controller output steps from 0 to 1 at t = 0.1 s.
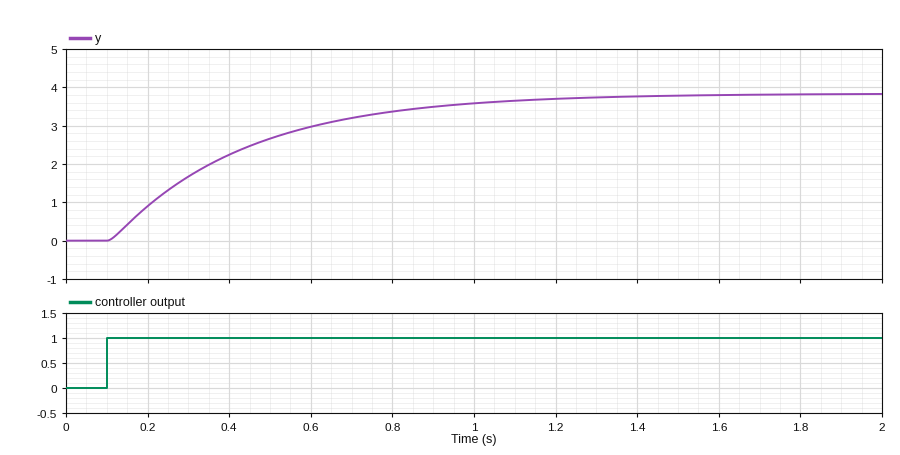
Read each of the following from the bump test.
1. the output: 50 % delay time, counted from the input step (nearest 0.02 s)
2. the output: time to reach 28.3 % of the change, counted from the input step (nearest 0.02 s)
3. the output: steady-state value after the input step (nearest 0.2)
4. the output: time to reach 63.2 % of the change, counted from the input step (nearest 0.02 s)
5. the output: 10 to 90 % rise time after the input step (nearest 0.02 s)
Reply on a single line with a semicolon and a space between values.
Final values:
0.24 s; 0.12 s; 3.8; 0.34 s; 0.72 s
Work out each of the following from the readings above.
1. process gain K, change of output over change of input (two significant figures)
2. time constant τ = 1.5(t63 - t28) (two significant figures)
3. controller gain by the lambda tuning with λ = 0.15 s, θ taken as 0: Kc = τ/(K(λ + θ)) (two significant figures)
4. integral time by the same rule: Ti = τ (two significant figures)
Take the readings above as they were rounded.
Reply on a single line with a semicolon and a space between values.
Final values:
3.8; 0.33 s; 0.58; 0.33 s
